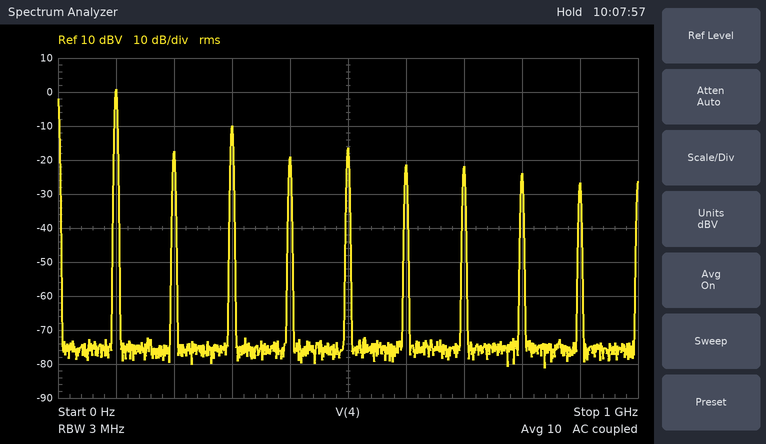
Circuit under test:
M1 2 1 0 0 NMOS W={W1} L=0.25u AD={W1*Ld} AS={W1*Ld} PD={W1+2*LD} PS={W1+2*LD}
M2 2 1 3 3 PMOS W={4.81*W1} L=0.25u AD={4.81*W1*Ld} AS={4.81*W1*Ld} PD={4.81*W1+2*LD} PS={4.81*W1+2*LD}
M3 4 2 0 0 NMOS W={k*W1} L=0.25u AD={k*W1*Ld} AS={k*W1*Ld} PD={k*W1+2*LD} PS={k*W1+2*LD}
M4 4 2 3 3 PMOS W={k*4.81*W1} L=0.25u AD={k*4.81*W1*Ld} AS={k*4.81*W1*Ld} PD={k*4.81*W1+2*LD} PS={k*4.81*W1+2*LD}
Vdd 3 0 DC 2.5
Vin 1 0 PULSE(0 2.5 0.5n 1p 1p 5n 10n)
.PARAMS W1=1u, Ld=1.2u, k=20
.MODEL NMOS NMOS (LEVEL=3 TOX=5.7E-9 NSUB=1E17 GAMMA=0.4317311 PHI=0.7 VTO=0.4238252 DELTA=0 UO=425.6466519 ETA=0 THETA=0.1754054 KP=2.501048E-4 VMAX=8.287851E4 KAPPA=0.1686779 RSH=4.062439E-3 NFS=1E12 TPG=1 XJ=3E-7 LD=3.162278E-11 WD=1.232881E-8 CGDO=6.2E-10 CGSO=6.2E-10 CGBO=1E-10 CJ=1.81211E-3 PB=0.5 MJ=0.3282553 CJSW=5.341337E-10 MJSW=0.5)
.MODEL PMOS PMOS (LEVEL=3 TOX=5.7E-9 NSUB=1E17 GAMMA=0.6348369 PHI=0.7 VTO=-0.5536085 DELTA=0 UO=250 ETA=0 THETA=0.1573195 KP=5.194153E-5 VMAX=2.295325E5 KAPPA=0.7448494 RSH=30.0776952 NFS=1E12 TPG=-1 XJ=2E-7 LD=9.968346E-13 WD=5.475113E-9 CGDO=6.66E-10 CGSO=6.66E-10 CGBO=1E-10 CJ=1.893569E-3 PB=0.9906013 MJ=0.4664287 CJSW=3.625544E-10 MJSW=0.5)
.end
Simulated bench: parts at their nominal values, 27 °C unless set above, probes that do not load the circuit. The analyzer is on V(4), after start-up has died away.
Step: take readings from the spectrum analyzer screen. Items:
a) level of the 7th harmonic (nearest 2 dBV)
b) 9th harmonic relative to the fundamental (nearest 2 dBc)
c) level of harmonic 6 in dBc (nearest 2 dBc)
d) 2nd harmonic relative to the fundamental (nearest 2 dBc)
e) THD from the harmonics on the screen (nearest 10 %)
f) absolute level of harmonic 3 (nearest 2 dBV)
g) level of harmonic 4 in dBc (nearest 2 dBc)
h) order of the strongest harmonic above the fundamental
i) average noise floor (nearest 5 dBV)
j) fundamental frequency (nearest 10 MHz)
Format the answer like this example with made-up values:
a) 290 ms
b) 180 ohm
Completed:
a) -22 dBV
b) -28 dBc
c) -22 dBc
d) -18 dBc
e) 40 %
f) -10 dBV
g) -20 dBc
h) 3
i) -75 dBV
j) 100 MHz
